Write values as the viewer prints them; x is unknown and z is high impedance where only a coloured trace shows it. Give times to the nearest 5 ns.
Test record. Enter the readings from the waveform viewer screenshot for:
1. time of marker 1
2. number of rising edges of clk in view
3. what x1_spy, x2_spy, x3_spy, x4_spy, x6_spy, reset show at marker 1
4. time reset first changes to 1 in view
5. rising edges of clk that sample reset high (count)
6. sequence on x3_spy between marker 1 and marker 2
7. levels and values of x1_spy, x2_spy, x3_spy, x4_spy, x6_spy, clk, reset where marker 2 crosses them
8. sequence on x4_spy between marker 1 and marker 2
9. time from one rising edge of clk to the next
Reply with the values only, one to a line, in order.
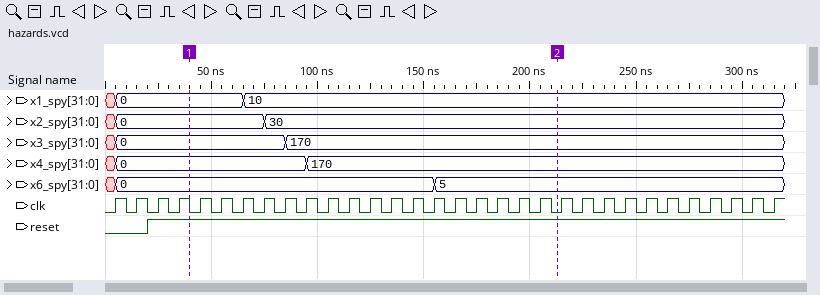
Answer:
40 ns
32
x1_spy=0, x2_spy=0, x3_spy=0, x4_spy=0, x6_spy=0, reset=1
20 ns
30
0, 170
x1_spy=10, x2_spy=30, x3_spy=170, x4_spy=170, x6_spy=5, clk=0, reset=1
0, 170
10 ns
